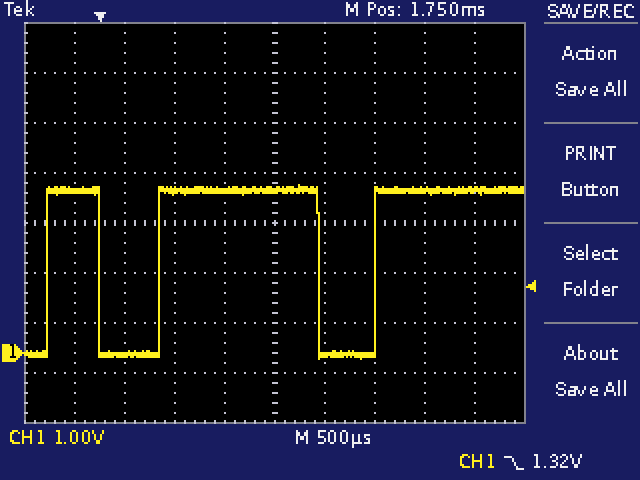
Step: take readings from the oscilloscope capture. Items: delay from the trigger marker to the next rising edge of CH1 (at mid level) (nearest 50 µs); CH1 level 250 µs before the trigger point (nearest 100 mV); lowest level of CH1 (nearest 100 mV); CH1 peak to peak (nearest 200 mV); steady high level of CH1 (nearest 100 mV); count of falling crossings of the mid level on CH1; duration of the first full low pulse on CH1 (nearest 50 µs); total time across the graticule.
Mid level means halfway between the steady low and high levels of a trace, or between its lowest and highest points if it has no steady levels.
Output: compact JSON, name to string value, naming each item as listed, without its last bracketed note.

{"delay from the trigger marker to the next rising edge of CH1 (at mid level)": "600 µs", "CH1 level 250 µs before the trigger point": "3.2 V", "lowest level of CH1": "-100 mV", "CH1 peak to peak": "3.4 V", "steady high level of CH1": "3.2 V", "count of falling crossings of the mid level on CH1": "2", "duration of the first full low pulse on CH1": "600 µs", "total time across the graticule": "5 ms"}
